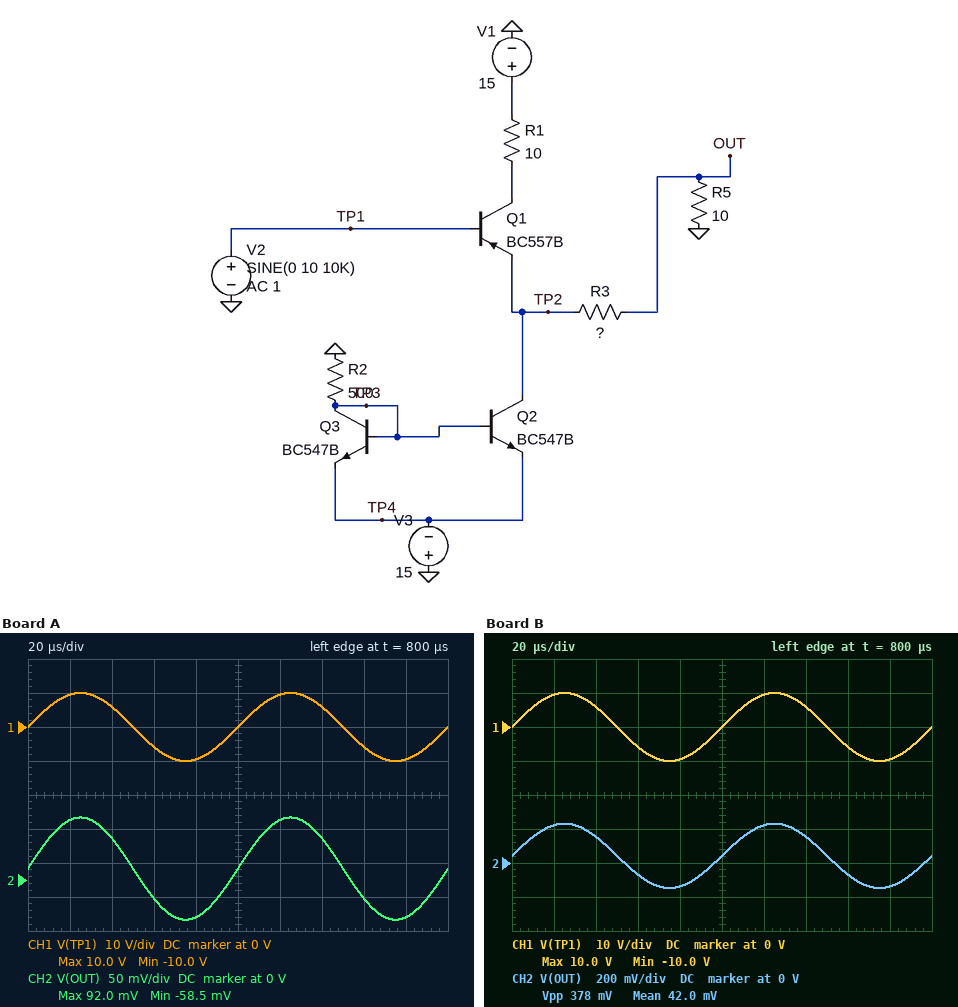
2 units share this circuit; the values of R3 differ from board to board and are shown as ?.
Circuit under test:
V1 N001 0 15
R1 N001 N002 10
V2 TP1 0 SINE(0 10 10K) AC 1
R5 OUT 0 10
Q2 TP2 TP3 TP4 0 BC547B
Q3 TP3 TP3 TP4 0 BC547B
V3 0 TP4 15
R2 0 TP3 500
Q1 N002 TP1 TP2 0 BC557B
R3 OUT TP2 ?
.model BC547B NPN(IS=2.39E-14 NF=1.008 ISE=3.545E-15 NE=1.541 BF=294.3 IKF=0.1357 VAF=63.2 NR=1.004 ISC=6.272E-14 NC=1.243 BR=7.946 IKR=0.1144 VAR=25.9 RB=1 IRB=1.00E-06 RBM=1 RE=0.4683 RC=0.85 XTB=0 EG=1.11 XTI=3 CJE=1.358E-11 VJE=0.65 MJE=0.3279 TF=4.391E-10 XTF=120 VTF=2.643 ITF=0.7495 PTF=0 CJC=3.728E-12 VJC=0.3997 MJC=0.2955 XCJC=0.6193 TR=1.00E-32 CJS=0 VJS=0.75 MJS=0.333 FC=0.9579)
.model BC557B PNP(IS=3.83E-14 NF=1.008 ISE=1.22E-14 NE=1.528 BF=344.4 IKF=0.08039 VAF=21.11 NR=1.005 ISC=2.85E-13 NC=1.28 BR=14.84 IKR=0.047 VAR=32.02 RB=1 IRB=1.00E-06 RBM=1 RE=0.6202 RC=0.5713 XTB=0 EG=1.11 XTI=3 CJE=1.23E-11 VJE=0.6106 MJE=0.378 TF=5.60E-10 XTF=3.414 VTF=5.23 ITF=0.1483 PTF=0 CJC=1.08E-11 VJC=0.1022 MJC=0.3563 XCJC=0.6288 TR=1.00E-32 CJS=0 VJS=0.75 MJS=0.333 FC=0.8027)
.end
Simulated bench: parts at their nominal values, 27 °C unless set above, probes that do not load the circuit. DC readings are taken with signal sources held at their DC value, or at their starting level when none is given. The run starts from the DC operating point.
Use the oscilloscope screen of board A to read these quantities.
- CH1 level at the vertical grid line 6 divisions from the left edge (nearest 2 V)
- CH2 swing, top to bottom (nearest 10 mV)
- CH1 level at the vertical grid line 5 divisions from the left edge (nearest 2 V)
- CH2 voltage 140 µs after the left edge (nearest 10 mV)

10 V
150 mV
0 V
60 mV
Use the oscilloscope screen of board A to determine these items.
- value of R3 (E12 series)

1.2 kΩ
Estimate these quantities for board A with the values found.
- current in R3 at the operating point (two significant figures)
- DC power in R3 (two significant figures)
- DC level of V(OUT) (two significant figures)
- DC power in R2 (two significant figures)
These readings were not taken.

1.7 mA
3.4 mW
17 mV
410 mW
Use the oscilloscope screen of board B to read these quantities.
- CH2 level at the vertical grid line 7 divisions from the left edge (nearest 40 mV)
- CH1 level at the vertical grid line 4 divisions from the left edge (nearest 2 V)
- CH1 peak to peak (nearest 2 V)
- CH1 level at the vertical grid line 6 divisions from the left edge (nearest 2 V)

160 mV
-10 V
20 V
10 V
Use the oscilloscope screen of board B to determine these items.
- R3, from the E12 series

470 Ω
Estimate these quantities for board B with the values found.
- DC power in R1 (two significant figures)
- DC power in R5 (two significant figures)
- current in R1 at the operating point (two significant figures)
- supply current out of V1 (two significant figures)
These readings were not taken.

15 W
180 µW
1.2 A
1.2 A
